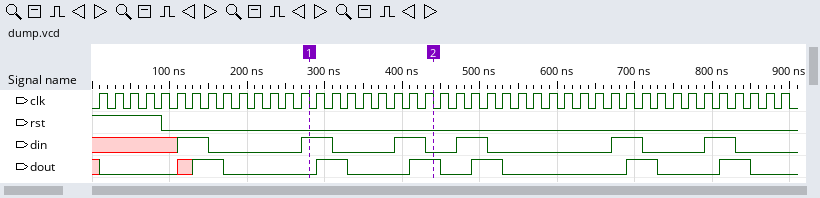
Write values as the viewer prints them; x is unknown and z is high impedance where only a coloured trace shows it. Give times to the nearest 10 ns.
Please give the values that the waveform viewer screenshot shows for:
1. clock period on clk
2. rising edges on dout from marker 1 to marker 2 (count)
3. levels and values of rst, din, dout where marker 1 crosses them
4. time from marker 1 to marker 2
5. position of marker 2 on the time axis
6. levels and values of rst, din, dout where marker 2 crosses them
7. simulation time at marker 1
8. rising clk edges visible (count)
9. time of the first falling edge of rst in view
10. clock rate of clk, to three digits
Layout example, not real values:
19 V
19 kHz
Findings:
20 ns
2
rst=0, din=1, dout=0
160 ns
440 ns
rst=0, din=0, dout=1
280 ns
45
90 ns
50.0 MHz
